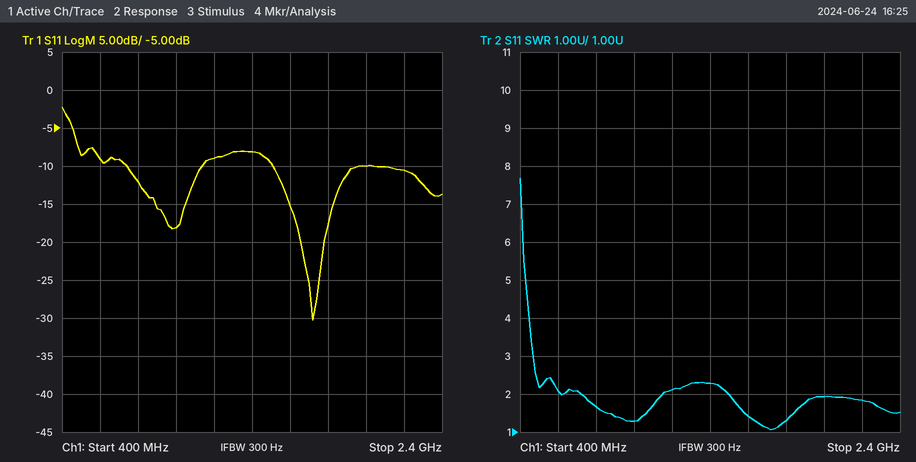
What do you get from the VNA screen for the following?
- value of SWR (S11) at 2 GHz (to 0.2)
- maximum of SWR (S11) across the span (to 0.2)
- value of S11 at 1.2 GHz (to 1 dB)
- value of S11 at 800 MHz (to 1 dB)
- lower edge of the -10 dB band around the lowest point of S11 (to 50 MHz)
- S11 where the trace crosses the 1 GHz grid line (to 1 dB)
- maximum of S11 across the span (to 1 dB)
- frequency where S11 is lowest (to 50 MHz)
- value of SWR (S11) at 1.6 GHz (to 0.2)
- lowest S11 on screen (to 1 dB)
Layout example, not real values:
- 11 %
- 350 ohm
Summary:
- 2.0
- 7.6
- -9 dB
- -12 dB
- 1.50 GHz
- -18 dB
- -2 dB
- 1.70 GHz
- 1.4
- -30 dB
